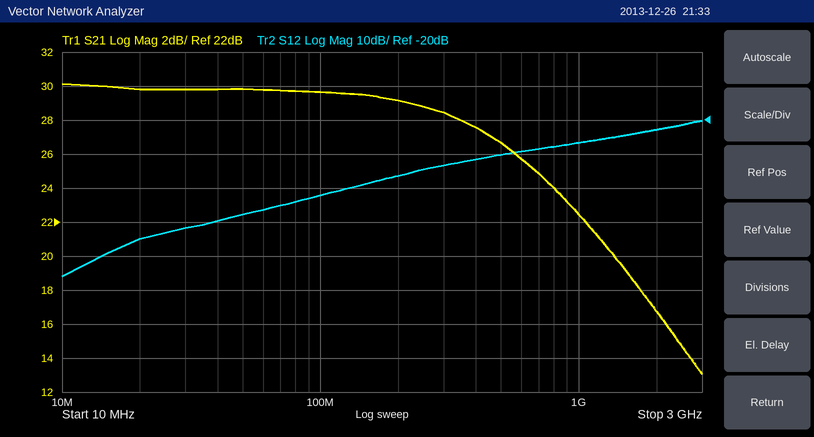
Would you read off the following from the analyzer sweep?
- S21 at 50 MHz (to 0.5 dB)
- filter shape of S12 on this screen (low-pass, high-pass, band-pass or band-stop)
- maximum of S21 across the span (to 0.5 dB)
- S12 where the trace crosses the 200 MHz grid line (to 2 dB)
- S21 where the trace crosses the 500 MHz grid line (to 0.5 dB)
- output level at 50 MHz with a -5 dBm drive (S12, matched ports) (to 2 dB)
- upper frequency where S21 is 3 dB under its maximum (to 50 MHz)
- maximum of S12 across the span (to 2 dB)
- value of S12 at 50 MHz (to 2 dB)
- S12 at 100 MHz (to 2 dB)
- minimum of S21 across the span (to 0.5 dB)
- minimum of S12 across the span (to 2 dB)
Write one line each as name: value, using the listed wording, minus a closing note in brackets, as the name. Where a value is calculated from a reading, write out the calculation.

S21 at 50 MHz: 30.0 dB
filter shape of S12 on this screen: high-pass
maximum of S21 across the span: 30.0 dB
S12 where the trace crosses the 200 MHz grid line: -36 dB
S21 where the trace crosses the 500 MHz grid line: 26.5 dB
output level at 50 MHz with a -5 dBm drive (S12, matched ports): -5 dBm + (-48 dB) = -52 dBm
upper frequency where S21 is 3 dB under its maximum: 450 MHz
maximum of S12 across the span: -20 dB
value of S12 at 50 MHz: -48 dB
S12 at 100 MHz: -42 dB
minimum of S21 across the span: 13.0 dB
minimum of S12 across the span: -66 dB
